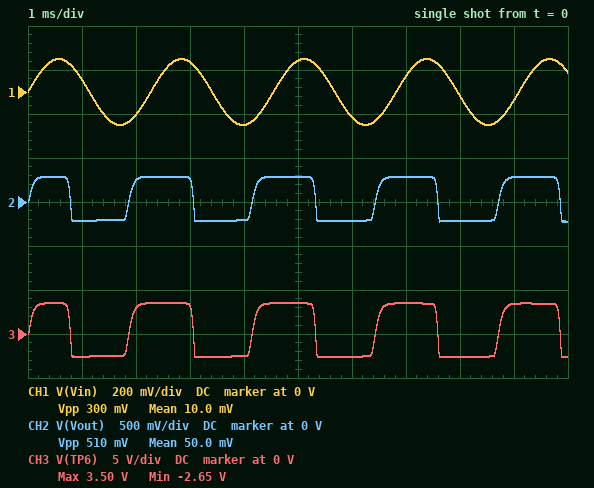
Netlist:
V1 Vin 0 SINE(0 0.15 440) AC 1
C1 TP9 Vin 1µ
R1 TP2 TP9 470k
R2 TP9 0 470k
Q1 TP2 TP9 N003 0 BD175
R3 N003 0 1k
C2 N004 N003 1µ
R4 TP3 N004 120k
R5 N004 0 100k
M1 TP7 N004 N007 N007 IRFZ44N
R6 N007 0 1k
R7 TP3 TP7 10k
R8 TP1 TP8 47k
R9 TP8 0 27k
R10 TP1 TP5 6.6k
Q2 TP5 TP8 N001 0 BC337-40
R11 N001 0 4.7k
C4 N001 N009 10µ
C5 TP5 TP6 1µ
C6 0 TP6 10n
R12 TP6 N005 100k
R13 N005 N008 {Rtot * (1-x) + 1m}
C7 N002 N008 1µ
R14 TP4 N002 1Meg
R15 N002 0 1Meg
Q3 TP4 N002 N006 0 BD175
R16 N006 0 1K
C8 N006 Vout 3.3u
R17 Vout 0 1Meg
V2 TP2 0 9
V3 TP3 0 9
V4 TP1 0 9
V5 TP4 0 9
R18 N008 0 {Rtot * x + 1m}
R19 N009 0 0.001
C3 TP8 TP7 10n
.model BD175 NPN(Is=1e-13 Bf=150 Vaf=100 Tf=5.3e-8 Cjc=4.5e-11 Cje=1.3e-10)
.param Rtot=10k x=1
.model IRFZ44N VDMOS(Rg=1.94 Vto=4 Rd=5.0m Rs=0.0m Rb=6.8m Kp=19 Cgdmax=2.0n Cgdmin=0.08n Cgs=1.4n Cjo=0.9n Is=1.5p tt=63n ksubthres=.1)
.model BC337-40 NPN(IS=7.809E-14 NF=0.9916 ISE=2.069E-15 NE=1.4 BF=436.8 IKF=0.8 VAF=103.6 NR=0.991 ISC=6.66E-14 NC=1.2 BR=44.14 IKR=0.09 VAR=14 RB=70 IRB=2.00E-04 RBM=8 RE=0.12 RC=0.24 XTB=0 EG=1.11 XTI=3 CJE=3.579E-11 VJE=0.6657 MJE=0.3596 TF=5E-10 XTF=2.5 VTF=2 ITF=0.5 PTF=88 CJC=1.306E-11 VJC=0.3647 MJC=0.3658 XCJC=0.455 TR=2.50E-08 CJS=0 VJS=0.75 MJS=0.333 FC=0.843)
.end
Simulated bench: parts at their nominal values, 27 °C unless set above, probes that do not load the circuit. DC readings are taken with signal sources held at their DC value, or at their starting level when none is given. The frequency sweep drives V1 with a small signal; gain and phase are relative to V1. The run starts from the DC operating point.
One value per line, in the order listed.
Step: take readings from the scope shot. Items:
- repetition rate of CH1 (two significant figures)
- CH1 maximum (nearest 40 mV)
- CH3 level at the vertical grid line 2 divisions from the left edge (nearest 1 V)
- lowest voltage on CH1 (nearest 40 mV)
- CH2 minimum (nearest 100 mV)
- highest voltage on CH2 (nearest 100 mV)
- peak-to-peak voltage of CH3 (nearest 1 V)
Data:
440 Hz
160 mV
3 V
-160 mV
-200 mV
300 mV
6 V
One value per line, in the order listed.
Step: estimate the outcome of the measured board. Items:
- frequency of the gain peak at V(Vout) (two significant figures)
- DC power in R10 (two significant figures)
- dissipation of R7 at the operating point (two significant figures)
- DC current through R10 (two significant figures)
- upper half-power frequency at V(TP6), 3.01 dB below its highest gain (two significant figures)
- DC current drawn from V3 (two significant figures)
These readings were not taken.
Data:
1.5 kHz
2.1 mW
1.3 mW
570 µA
4.0 kHz
410 µA
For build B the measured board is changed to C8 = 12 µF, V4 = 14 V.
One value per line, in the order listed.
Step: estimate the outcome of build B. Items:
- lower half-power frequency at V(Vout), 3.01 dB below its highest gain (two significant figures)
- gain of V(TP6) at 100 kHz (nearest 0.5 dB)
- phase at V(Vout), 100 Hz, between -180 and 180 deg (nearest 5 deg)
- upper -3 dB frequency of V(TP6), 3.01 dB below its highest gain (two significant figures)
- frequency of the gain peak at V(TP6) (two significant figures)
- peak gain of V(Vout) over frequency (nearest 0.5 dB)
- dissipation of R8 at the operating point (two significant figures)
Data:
660 Hz
20.5 dB
145 deg
4.3 kHz
1.7 kHz
32.5 dB
1.7 mW
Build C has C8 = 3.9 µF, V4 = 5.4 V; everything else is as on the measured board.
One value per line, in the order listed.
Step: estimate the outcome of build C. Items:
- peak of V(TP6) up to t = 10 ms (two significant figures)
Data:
1.8 V
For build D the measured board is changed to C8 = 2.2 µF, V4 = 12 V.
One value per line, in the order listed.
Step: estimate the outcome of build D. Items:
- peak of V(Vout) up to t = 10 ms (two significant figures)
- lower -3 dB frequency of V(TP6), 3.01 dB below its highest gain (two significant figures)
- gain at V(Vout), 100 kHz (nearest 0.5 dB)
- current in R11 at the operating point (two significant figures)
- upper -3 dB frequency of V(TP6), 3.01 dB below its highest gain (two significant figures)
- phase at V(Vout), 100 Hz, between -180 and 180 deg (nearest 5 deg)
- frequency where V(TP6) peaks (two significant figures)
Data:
400 mV
640 Hz
-3.0 dB
800 µA
4.2 kHz
145 deg
1.6 kHz
